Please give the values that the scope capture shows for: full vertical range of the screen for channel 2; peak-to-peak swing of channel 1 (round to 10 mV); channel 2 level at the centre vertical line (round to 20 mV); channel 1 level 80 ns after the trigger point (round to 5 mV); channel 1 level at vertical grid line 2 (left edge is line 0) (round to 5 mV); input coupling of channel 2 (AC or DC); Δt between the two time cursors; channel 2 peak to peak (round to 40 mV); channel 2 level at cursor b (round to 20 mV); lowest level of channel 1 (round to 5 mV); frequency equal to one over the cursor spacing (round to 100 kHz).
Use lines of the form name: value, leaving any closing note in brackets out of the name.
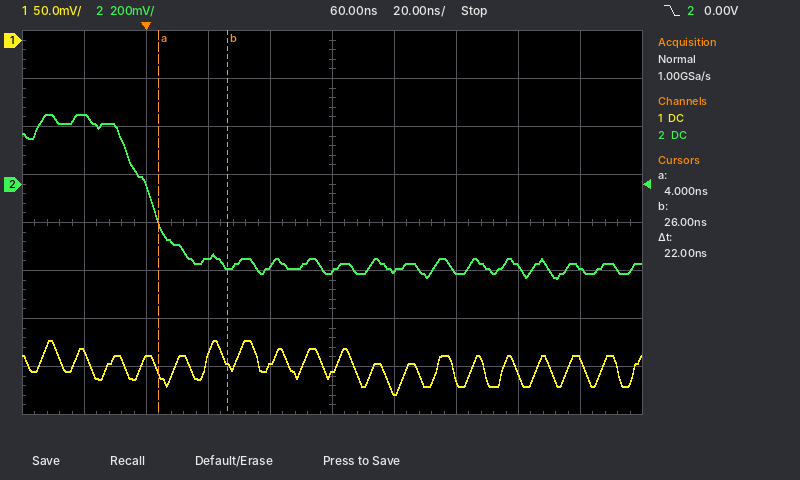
full vertical range of the screen for channel 2: 1.6 V
peak-to-peak swing of channel 1: 60 mV
channel 2 level at the centre vertical line: -360 mV
channel 1 level 80 ns after the trigger point: -365 mV
channel 1 level at vertical grid line 2 (left edge is line 0): -330 mV
input coupling of channel 2: DC
Δt between the two time cursors: 22 ns
channel 2 peak to peak: 680 mV
channel 2 level at cursor b: -340 mV
lowest level of channel 1: -370 mV
frequency equal to one over the cursor spacing: 45.5 MHz
